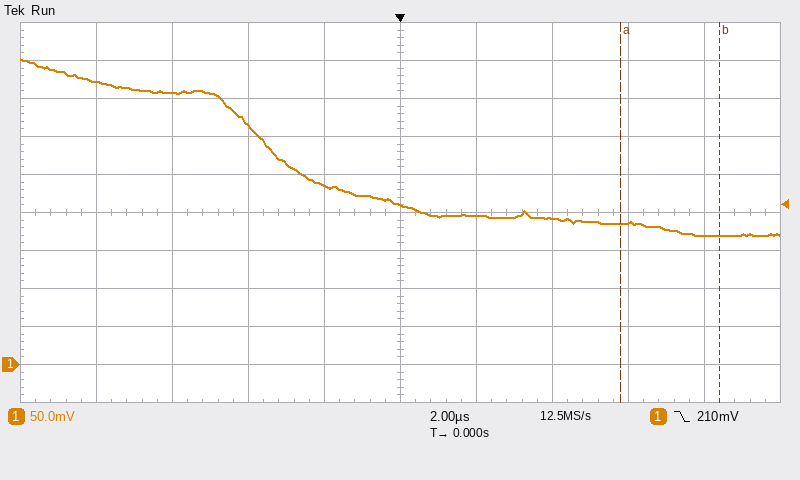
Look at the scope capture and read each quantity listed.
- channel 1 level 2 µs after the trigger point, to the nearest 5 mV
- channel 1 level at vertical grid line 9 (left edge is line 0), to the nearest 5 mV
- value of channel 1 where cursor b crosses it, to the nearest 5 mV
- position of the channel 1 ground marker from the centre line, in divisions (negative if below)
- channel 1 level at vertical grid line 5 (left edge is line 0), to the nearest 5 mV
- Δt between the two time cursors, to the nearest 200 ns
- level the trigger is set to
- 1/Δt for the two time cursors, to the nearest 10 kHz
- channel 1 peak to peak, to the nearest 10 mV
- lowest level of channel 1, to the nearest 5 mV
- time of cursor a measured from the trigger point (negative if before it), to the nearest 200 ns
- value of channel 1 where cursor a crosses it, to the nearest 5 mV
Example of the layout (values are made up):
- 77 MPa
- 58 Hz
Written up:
- 195 mV
- 170 mV
- 170 mV
- -4.0 div
- 210 mV
- 2.6 µs
- 210 mV
- 380 kHz
- 230 mV
- 170 mV
- +5.8 µs
- 185 mV
